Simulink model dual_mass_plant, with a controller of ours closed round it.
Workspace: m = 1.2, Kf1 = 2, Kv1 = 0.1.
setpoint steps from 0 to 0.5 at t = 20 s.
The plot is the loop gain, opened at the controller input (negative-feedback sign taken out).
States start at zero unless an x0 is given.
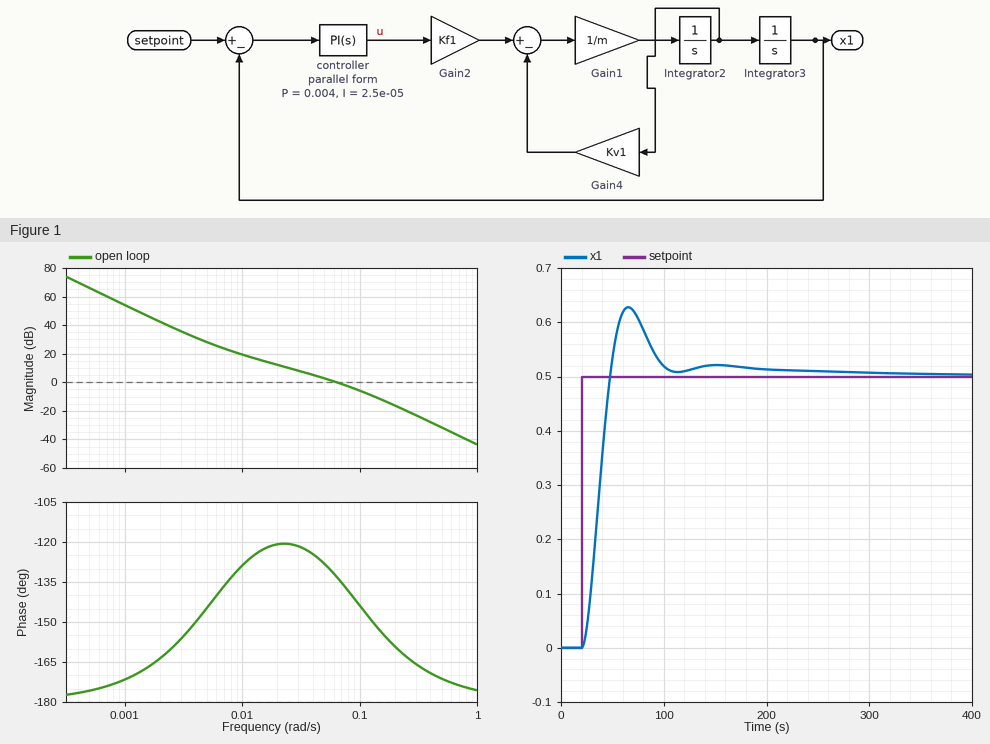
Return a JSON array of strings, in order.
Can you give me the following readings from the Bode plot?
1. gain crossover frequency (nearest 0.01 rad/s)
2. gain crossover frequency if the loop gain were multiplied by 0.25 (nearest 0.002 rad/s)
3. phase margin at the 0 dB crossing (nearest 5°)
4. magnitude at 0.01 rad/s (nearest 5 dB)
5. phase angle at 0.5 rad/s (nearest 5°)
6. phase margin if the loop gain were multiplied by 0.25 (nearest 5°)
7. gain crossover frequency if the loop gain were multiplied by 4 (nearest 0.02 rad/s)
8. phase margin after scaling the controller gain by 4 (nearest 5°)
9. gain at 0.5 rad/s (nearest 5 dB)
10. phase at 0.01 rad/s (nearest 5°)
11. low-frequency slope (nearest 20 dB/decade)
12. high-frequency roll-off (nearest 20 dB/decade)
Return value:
["0.06 rad/s", "0.020 rad/s", "45°", "20 dB", "-170°", "60°", "0.16 rad/s", "25°", "-30 dB", "-130°", "-40 dB/decade", "-40 dB/decade"]
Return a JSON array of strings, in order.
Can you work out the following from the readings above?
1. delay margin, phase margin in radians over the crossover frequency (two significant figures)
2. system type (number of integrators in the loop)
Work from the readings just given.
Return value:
["13 s", "2"]
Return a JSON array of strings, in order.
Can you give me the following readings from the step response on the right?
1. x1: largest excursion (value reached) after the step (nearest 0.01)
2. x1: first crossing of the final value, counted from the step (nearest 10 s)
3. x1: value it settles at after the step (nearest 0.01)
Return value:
["0.63", "30 s", "0.50"]
